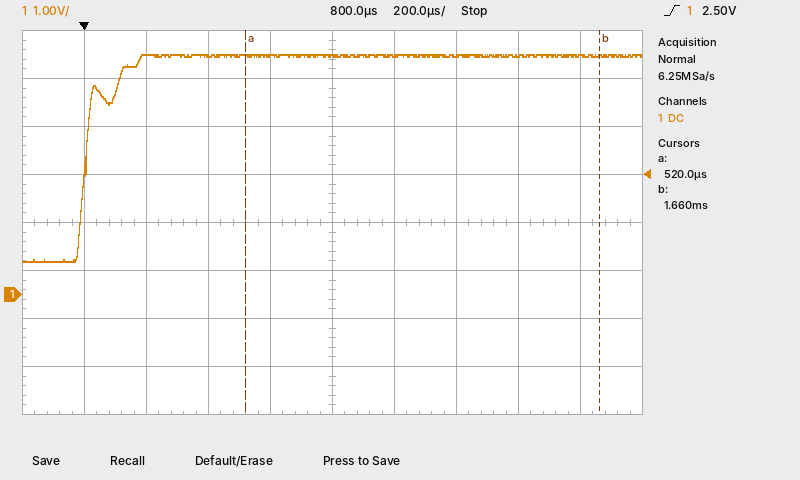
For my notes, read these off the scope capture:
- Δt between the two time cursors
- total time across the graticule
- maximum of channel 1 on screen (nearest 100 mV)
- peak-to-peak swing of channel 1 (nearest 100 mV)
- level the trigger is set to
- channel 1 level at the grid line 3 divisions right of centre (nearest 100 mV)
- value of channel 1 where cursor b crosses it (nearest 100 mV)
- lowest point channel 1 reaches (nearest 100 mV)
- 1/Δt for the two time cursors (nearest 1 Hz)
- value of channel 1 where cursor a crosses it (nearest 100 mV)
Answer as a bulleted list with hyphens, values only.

- 1.14 ms
- 2 ms
- 5.0 V
- 4.3 V
- 2.50 V
- 5.0 V
- 5.0 V
- 700 mV
- 877 Hz
- 5.0 V
